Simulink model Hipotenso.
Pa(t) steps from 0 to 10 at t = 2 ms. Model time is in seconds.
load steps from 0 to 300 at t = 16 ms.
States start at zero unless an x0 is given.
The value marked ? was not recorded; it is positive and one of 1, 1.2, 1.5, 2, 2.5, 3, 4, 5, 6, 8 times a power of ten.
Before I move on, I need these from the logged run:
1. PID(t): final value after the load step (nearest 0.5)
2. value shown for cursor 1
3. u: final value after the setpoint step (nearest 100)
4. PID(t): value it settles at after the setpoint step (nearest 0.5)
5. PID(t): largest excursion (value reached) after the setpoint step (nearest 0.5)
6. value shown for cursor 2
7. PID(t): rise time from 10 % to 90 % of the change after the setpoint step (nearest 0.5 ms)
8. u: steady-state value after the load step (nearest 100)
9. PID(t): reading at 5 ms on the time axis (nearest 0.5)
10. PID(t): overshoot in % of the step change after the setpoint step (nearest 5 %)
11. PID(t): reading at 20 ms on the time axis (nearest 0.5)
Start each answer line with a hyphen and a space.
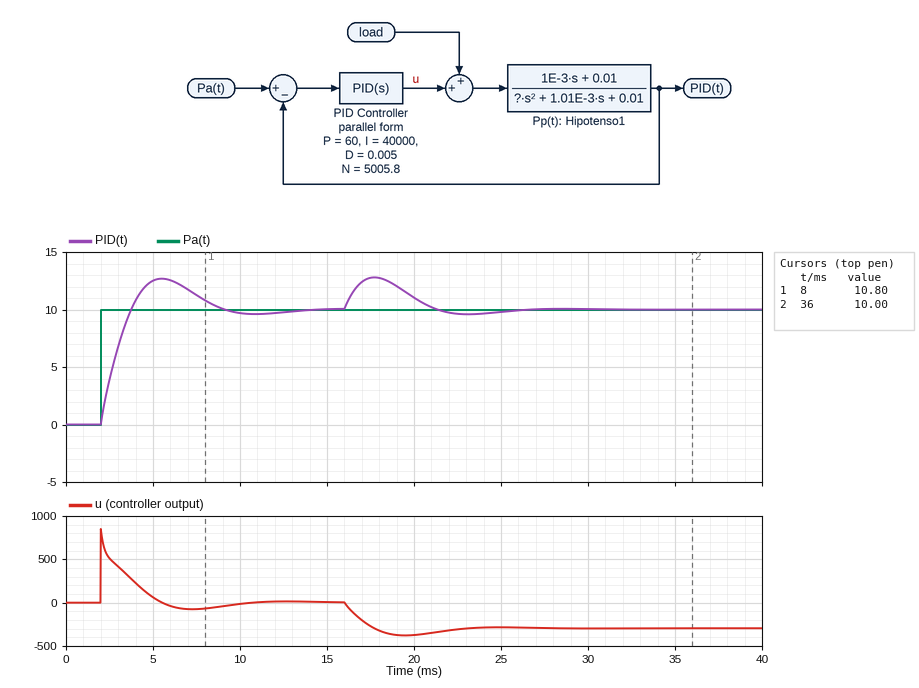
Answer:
- 10.0
- 10.80
- 0
- 10.0
- 12.5
- 10.00
- 1.5 ms
- -300
- 12.5
- 25 %
- 11.0
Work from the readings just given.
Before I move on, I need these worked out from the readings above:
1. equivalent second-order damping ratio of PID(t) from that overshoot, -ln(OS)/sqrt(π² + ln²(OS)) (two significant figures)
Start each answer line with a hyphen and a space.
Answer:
- 0.40
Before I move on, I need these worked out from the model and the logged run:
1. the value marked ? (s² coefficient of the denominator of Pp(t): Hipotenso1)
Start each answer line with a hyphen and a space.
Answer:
- 8e-05
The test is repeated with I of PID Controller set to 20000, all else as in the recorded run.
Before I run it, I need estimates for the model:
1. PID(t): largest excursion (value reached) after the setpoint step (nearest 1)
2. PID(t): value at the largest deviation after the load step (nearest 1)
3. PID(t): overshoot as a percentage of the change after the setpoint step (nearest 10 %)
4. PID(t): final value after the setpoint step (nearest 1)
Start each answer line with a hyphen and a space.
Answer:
- 12
- 13
- 20 %
- 10
